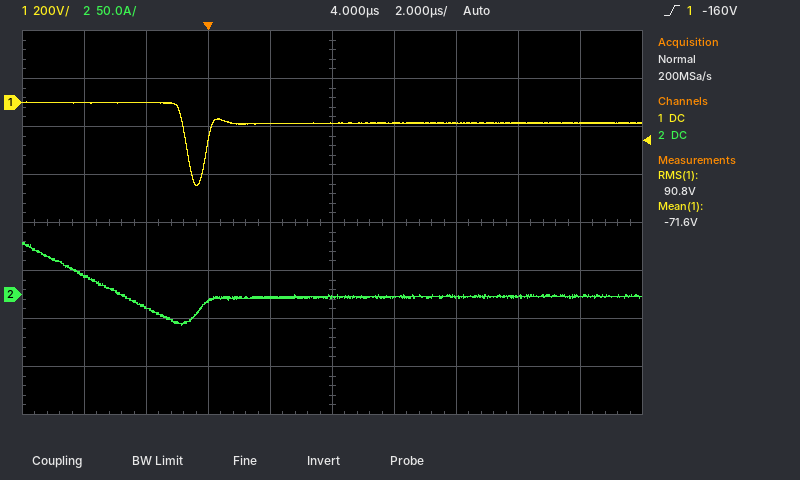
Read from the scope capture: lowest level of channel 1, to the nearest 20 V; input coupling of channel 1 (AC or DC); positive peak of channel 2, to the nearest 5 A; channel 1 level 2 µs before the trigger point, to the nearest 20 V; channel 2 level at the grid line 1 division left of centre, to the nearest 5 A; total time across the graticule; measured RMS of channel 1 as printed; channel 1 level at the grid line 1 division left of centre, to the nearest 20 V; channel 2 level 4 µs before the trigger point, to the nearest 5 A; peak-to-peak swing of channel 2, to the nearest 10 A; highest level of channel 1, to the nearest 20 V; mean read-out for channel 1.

-340 V
DC
55 A
0 V
-5 A
20 µs
90.8 V
-80 V
20 A
90 A
0 V
-71.6 V
